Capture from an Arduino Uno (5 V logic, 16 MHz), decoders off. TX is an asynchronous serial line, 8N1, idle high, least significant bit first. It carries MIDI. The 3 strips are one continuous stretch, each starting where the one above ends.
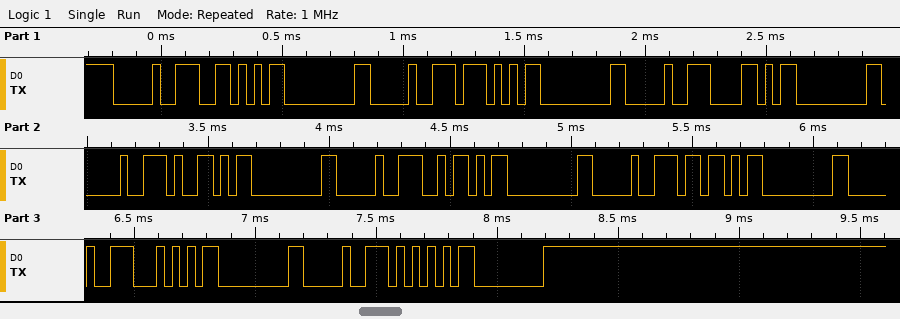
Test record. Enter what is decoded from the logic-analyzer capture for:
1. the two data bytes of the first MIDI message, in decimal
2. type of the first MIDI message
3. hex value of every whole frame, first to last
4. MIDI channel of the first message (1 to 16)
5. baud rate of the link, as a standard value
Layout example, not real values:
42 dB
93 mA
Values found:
86, 0
Note On
90 56 00 90 57 00 90 58 00 90 59 00 90 5A 00 90 5B 00 90 54 00 90 55 00
1
31250 baud
